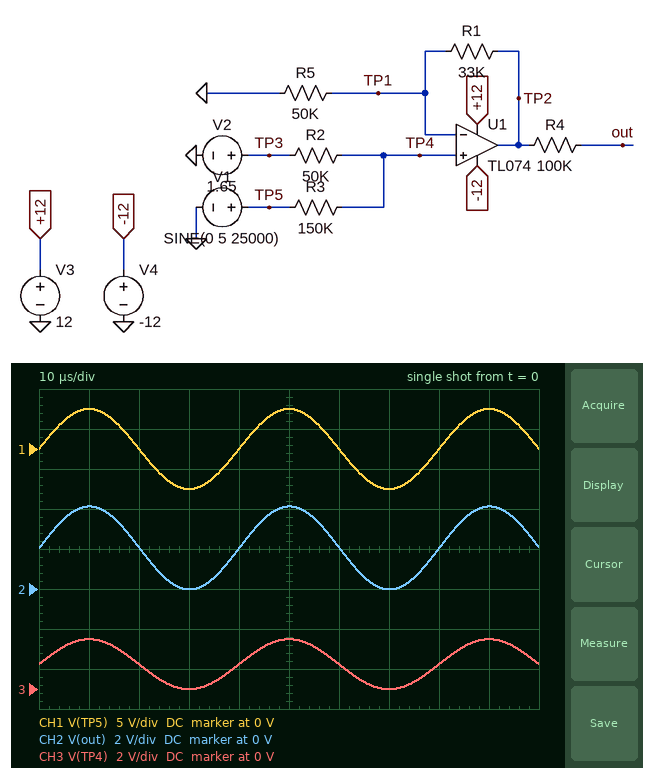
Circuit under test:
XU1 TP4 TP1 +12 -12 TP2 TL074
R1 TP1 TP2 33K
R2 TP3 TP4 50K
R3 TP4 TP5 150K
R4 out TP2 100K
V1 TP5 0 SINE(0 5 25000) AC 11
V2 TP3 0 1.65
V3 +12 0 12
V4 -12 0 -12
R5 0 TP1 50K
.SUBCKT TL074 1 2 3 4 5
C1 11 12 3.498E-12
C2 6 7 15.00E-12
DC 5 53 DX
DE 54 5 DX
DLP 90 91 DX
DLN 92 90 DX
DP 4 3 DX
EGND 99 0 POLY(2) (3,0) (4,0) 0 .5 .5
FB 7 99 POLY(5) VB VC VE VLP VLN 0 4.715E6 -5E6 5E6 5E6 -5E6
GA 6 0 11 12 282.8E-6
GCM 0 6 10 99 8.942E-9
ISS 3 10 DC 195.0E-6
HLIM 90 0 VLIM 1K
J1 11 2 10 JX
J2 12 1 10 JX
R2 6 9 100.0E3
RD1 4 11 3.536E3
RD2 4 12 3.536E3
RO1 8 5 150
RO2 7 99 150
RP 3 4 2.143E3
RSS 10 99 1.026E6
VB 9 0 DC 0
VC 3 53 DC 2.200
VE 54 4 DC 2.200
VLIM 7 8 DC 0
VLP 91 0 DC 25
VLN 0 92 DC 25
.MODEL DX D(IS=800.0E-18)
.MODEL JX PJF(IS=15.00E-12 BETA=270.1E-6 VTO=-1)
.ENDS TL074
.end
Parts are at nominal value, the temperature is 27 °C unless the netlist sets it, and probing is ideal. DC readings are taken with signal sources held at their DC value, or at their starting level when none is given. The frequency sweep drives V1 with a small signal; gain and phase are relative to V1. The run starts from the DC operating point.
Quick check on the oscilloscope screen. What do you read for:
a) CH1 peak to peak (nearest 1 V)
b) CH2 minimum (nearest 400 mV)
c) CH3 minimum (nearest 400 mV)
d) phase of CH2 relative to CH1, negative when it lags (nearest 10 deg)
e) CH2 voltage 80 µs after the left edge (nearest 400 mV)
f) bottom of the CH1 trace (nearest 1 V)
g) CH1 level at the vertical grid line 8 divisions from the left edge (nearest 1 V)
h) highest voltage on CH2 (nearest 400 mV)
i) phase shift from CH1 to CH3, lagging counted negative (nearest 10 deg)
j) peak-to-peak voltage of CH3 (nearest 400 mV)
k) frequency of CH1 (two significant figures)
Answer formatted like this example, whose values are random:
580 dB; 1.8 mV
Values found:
10 V; 0 V; 0 V; 0 deg; 2.0 V; -5 V; 0 V; 4.0 V; 0 deg; 2.4 V; 25 kHz
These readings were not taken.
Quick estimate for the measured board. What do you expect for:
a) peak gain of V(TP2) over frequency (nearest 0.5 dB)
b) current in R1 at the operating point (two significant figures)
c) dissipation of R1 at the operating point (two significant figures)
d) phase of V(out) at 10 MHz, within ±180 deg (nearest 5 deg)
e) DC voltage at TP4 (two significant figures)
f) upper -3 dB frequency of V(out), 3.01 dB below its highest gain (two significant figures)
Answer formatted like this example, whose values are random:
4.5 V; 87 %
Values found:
-7.5 dB; 25 µA; 20 µW; -145 deg; 1.2 V; 2.8 MHz
